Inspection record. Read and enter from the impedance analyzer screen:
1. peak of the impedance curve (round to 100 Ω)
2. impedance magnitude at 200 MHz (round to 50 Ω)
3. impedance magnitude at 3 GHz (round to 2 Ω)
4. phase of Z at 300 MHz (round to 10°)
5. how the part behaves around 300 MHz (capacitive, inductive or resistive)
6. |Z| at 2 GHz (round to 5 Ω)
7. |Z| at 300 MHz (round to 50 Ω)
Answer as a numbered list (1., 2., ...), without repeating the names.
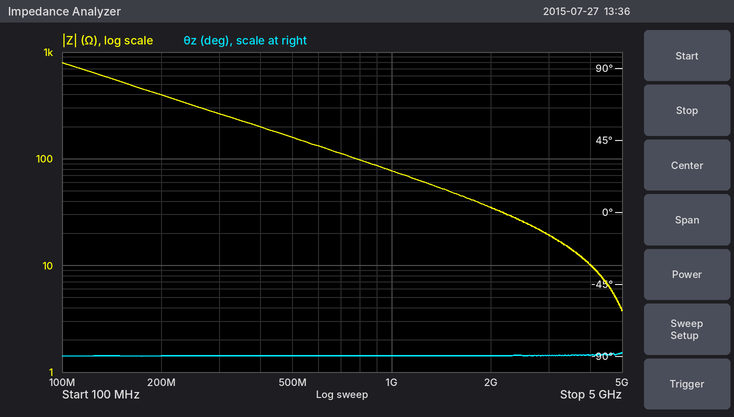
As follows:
1. 800 Ω
2. 400 Ω
3. 20 Ω
4. -90°
5. capacitive
6. 35 Ω
7. 250 Ω
